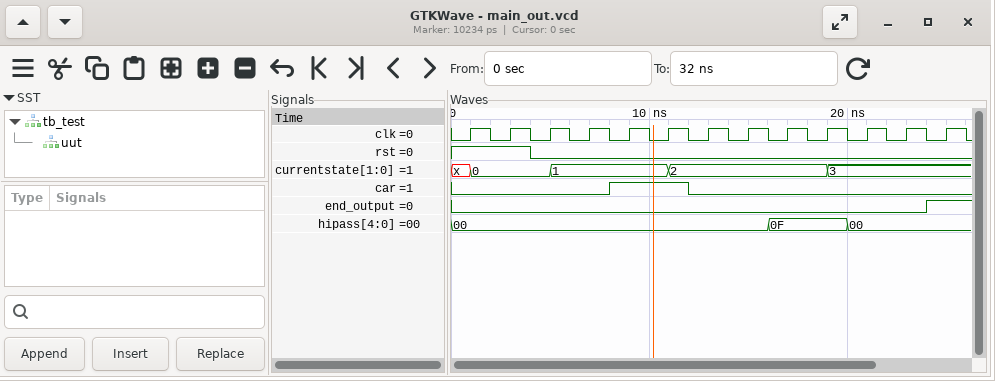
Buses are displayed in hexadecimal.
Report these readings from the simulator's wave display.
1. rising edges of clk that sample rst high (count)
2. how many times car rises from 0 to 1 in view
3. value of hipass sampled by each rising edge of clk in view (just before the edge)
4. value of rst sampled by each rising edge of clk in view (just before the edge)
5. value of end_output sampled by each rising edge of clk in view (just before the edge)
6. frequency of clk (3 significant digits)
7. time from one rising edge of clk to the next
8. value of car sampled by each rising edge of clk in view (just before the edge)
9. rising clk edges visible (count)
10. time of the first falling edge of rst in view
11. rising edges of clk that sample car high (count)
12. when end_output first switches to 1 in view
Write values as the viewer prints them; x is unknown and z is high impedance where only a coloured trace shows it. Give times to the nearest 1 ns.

2
1
00, 00, 00, 00, 00, 00, 00, 00, 0F, 0F, 00, 00, 00
1 1 0 0 0 0 0 0 0 0 0 0 0
0 0 0 0 0 0 0 0 0 0 0 0 1
500 MHz
2 ns
0 0 0 0 1 1 0 0 0 0 0 0 0
13
4 ns
2
24 ns
